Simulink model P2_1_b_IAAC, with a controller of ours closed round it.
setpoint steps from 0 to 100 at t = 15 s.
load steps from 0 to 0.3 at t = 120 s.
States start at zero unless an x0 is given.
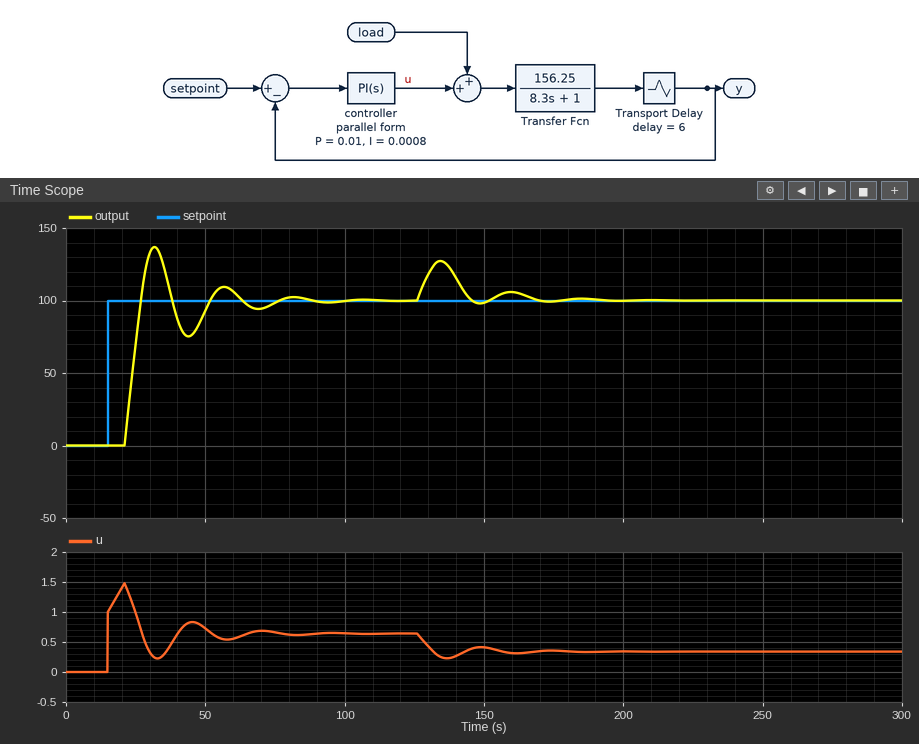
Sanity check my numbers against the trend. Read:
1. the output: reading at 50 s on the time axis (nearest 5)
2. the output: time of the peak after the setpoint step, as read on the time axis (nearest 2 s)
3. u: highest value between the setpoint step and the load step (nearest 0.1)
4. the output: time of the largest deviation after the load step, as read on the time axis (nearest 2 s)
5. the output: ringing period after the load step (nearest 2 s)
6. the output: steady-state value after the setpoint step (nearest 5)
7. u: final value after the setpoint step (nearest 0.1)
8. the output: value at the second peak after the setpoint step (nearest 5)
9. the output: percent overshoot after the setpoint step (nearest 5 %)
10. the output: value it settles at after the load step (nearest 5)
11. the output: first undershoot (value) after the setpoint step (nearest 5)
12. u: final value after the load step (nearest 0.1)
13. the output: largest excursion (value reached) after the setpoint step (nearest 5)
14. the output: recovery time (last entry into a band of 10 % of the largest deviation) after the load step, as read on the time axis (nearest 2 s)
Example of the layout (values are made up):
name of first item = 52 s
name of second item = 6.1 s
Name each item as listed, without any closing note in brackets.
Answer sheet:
the output: reading at 50 s on the time axis = 95
the output: time of the peak after the setpoint step, as read on the time axis = 32 s
u: highest value between the setpoint step and the load step = 1.5
the output: time of the largest deviation after the load step, as read on the time axis = 134 s
the output: ringing period after the load step = 26 s
the output: steady-state value after the setpoint step = 100
u: final value after the setpoint step = 0.6
the output: value at the second peak after the setpoint step = 110
the output: percent overshoot after the setpoint step = 35 %
the output: value it settles at after the load step = 100
the output: first undershoot (value) after the setpoint step = 75
u: final value after the load step = 0.3
the output: largest excursion (value reached) after the setpoint step = 135
the output: recovery time (last entry into a band of 10 % of the largest deviation) after the load step, as read on the time axis = 166 s
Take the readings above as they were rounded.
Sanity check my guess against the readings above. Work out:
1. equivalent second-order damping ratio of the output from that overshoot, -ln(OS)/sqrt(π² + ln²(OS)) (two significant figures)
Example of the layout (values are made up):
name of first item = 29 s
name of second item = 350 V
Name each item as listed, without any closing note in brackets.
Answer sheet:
equivalent second-order damping ratio of the output from that overshoot, -ln(OS)/sqrt(π² + ln²(OS)) = 0.32
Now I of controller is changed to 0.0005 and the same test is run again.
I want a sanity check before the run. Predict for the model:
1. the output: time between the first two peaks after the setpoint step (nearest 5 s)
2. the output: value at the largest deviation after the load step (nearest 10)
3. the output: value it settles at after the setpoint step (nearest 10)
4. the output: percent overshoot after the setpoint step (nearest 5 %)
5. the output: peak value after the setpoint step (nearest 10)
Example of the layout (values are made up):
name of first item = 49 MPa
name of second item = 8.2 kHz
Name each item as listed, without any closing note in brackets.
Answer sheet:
the output: time between the first two peaks after the setpoint step = 25 s
the output: value at the largest deviation after the load step = 130
the output: value it settles at after the setpoint step = 100
the output: percent overshoot after the setpoint step = 20 %
the output: peak value after the setpoint step = 120
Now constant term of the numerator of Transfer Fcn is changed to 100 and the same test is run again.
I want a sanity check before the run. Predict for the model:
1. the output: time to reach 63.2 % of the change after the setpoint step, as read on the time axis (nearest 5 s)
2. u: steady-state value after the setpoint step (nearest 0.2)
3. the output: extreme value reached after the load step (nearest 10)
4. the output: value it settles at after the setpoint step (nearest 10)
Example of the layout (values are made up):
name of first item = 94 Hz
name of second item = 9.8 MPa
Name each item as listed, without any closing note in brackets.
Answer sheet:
the output: time to reach 63.2 % of the change after the setpoint step, as read on the time axis = 25 s
u: steady-state value after the setpoint step = 1.0
the output: extreme value reached after the load step = 120
the output: value it settles at after the setpoint step = 100
